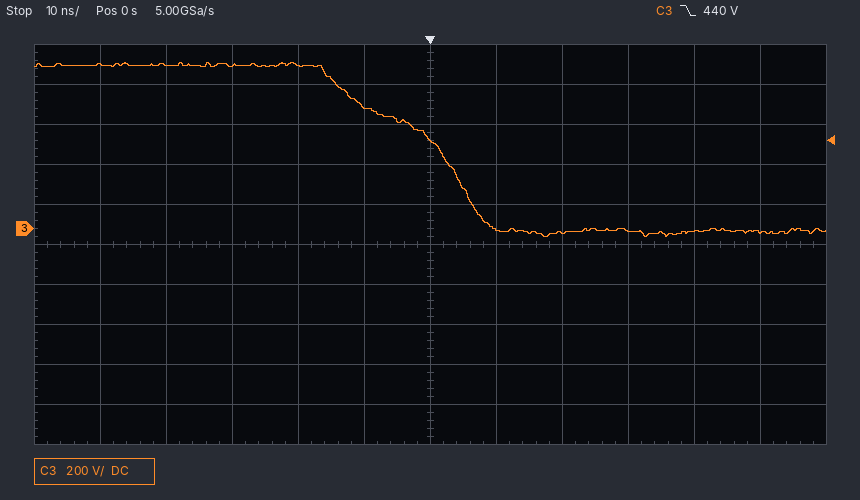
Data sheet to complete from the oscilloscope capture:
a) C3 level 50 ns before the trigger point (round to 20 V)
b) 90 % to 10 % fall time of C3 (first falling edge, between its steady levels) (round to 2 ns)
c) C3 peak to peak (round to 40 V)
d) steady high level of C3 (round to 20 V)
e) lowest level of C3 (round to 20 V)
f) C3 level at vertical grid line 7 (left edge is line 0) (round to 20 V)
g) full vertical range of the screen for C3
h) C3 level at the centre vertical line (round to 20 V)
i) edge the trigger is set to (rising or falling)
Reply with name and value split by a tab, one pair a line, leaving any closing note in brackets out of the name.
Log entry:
C3 level 50 ns before the trigger point	820 V
90 % to 10 % fall time of C3 (first falling edge, between its steady levels)	22 ns
C3 peak to peak	880 V
steady high level of C3	820 V
lowest level of C3	-40 V
C3 level at vertical grid line 7 (left edge is line 0)	0 V
full vertical range of the screen for C3	2 kV
C3 level at the centre vertical line	440 V
edge the trigger is set to	falling
